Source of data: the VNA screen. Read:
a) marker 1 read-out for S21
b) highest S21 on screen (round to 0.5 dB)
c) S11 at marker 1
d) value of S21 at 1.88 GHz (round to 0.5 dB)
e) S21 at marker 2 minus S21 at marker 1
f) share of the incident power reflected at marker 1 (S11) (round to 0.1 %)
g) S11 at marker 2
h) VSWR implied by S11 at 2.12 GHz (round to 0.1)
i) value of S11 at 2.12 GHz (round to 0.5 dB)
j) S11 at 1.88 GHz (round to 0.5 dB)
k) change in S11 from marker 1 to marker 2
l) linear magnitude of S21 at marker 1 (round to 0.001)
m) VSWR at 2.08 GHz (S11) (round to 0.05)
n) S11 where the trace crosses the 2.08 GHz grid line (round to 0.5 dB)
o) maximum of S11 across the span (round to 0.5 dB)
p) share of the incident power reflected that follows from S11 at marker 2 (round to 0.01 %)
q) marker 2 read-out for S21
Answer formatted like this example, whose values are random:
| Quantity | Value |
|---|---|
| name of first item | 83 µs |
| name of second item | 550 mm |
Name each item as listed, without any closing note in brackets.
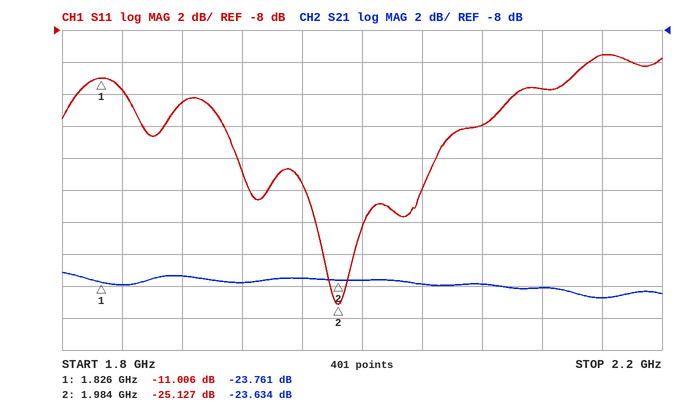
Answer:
| Quantity | Value |
|---|---|
| marker 1 read-out for S21 | -23.761 dB |
| highest S21 on screen | -23.0 dB |
| S11 at marker 1 | -11.006 dB |
| value of S21 at 1.88 GHz | -23.5 dB |
| S21 at marker 2 minus S21 at marker 1 | 0.127 dB |
| share of the incident power reflected at marker 1 (S11) | 7.9 % |
| S11 at marker 2 | -25.127 dB |
| VSWR implied by S11 at 2.12 GHz | 1.7 |
| value of S11 at 2.12 GHz | -11.5 dB |
| S11 at 1.88 GHz | -12.5 dB |
| change in S11 from marker 1 to marker 2 | -14.121 dB |
| linear magnitude of S21 at marker 1 | 0.065 |
| VSWR at 2.08 GHz (S11) | 1.50 |
| S11 where the trace crosses the 2.08 GHz grid line | -14.0 dB |
| maximum of S11 across the span | -9.5 dB |
| share of the incident power reflected that follows from S11 at marker 2 | 0.31 % |
| marker 2 read-out for S21 | -23.634 dB |
